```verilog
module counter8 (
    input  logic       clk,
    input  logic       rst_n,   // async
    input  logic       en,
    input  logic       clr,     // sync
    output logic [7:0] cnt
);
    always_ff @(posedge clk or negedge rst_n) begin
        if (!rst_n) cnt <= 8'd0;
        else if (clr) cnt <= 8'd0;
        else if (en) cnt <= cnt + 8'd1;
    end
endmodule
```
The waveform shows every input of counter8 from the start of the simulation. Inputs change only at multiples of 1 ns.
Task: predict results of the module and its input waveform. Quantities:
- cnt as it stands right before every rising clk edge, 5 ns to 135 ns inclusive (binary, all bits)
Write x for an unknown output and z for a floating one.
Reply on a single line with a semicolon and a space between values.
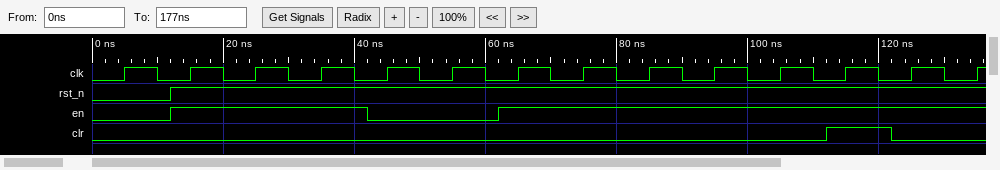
00000000, 00000000, 00000001, 00000010, 00000011, 00000011, 00000011, 00000100, 00000101, 00000110, 00000111, 00001000, 00000000, 00000001
